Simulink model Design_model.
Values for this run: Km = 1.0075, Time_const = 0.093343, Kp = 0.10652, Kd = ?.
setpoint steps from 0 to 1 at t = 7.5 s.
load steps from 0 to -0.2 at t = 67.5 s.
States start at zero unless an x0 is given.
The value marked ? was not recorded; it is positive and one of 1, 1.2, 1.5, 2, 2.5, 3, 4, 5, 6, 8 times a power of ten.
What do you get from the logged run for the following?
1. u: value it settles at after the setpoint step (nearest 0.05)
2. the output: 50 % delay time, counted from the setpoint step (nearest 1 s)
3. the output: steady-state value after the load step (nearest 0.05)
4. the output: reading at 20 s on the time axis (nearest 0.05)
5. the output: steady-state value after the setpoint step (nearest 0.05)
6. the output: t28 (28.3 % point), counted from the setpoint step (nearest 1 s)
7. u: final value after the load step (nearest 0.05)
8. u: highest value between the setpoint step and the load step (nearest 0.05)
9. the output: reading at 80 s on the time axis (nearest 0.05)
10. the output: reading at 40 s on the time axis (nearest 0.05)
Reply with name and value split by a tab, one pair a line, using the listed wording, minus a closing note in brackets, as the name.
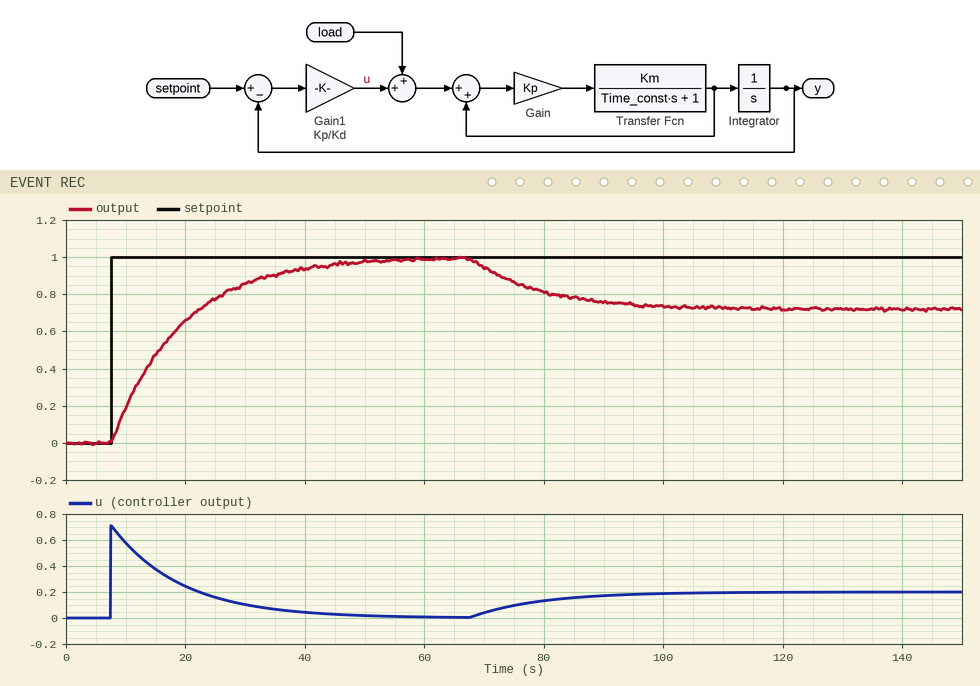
u: value it settles at after the setpoint step	0.00
the output: 50 % delay time, counted from the setpoint step	8 s
the output: steady-state value after the load step	0.70
the output: reading at 20 s on the time axis	0.65
the output: steady-state value after the setpoint step	1.00
the output: t28 (28.3 % point), counted from the setpoint step	4 s
u: final value after the load step	0.20
u: highest value between the setpoint step and the load step	0.70
the output: reading at 80 s on the time axis	0.80
the output: reading at 40 s on the time axis	0.95
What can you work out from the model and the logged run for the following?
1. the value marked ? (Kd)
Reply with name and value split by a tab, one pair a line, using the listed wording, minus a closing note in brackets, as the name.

the value marked ?	0.15
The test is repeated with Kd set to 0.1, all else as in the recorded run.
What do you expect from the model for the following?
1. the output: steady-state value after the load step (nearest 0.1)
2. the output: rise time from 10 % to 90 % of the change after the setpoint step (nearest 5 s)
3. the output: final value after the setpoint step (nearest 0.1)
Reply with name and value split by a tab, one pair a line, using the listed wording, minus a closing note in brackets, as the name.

the output: steady-state value after the load step	0.8
the output: rise time from 10 % to 90 % of the change after the setpoint step	15 s
the output: final value after the setpoint step	1.0
